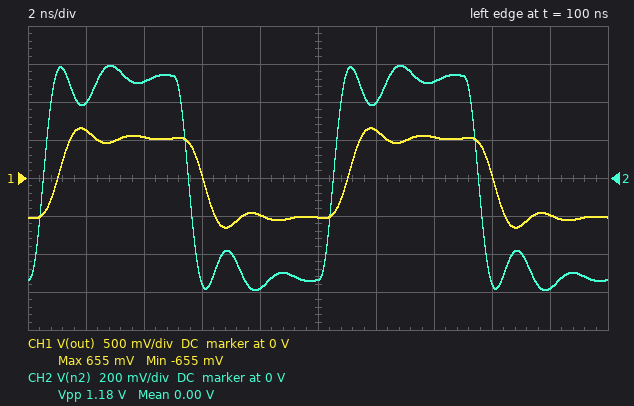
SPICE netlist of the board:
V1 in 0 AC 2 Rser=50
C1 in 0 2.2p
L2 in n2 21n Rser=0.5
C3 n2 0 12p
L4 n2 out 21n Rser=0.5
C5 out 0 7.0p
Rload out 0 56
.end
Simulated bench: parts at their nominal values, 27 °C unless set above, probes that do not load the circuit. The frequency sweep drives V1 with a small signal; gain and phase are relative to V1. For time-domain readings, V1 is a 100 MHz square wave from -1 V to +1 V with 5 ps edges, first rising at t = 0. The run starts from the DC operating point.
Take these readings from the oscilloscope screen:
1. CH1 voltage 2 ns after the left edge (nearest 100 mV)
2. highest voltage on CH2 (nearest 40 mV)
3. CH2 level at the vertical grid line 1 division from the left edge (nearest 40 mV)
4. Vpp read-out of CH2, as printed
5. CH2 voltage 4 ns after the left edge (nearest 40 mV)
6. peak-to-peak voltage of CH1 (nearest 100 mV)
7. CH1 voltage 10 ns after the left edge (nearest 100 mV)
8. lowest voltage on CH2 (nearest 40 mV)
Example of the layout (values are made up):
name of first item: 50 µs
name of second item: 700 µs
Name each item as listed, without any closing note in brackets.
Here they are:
CH1 voltage 2 ns after the left edge: 600 mV
highest voltage on CH2: 600 mV
CH2 level at the vertical grid line 1 division from the left edge: 400 mV
Vpp read-out of CH2, as printed: 1.18 V
CH2 voltage 4 ns after the left edge: 520 mV
peak-to-peak voltage of CH1: 1.3 V
CH1 voltage 10 ns after the left edge: -500 mV
lowest voltage on CH2: -600 mV
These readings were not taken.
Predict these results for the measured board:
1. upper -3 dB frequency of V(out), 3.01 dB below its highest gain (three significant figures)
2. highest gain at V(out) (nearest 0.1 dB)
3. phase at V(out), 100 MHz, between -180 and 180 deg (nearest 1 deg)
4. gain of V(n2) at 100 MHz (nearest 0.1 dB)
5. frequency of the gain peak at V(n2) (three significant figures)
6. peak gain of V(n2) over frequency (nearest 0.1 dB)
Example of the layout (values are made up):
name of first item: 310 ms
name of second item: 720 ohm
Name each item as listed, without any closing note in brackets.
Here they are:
upper -3 dB frequency of V(out), 3.01 dB below its highest gain: 574 MHz
highest gain at V(out): -5.6 dB
phase at V(out), 100 MHz, between -180 and 180 deg: -35 deg
gain of V(n2) at 100 MHz: -5.8 dB
frequency of the gain peak at V(n2): 532 MHz
peak gain of V(n2) over frequency: -3.9 dB
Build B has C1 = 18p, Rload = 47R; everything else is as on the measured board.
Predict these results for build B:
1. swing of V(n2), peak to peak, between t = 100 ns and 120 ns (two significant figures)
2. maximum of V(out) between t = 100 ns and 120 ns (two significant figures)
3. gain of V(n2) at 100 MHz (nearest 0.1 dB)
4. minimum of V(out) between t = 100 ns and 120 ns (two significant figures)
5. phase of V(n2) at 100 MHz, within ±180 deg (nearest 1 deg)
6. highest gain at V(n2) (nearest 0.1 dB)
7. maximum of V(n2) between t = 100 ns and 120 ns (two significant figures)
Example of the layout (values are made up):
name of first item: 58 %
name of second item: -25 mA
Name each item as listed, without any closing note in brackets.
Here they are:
swing of V(n2), peak to peak, between t = 100 ns and 120 ns: 1.1 V
maximum of V(out) between t = 100 ns and 120 ns: 560 mV
gain of V(n2) at 100 MHz: -6.7 dB
minimum of V(out) between t = 100 ns and 120 ns: -560 mV
phase of V(n2) at 100 MHz, within ±180 deg: -31 deg
highest gain at V(n2): -5.3 dB
maximum of V(n2) between t = 100 ns and 120 ns: 540 mV
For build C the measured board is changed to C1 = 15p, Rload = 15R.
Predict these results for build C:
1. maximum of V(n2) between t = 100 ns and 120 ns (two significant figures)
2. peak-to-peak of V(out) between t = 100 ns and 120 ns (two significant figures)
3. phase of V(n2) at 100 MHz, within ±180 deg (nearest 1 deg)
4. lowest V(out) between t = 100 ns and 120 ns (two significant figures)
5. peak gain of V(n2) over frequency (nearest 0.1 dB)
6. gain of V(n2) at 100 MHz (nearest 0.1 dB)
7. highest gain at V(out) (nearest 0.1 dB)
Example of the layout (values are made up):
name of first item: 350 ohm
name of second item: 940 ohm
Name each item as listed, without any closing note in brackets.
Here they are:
maximum of V(n2) between t = 100 ns and 120 ns: 830 mV
peak-to-peak of V(out) between t = 100 ns and 120 ns: 620 mV
phase of V(n2) at 100 MHz, within ±180 deg: 1 deg
lowest V(out) between t = 100 ns and 120 ns: -310 mV
peak gain of V(n2) over frequency: 1.1 dB
gain of V(n2) at 100 MHz: -9.8 dB
highest gain at V(out): -11.7 dB
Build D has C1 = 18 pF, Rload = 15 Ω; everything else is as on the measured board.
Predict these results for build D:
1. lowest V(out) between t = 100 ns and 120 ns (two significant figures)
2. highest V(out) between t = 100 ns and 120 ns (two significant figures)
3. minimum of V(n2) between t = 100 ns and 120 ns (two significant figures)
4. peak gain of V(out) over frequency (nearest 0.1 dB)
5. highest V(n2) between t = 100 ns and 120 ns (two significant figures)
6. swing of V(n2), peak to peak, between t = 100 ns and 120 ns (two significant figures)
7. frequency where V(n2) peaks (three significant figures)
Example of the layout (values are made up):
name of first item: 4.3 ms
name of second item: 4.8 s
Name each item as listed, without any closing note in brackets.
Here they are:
lowest V(out) between t = 100 ns and 120 ns: -310 mV
highest V(out) between t = 100 ns and 120 ns: 310 mV
minimum of V(n2) between t = 100 ns and 120 ns: -790 mV
peak gain of V(out) over frequency: -11.8 dB
highest V(n2) between t = 100 ns and 120 ns: 790 mV
swing of V(n2), peak to peak, between t = 100 ns and 120 ns: 1.6 V
frequency where V(n2) peaks: 486 MHz
